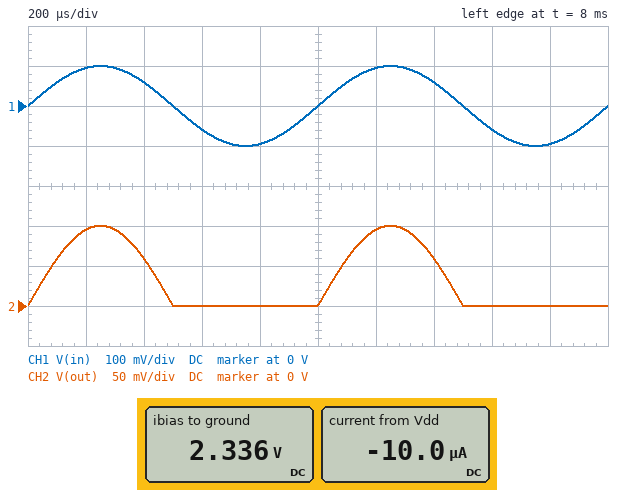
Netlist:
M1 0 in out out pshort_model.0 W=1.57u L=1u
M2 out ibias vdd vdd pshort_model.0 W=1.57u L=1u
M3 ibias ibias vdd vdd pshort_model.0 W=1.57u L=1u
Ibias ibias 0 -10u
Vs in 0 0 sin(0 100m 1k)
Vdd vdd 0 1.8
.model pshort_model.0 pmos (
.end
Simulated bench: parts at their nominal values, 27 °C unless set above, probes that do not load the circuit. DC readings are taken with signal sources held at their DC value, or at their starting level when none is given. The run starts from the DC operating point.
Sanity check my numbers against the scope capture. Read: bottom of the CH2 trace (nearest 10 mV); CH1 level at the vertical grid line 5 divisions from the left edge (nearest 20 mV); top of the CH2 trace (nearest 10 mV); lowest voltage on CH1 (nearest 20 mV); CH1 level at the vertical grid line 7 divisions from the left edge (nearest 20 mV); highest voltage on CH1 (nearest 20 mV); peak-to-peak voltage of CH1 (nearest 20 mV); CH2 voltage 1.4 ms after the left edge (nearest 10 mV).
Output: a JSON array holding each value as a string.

["0 V", "0 V", "100 mV", "-100 mV", "60 mV", "100 mV", "200 mV", "60 mV"]
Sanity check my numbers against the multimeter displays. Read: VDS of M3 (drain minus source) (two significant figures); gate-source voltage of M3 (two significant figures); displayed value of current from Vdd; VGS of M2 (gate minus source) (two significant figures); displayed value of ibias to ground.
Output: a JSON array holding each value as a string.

["540 mV", "540 mV", "-10.0 µA", "540 mV", "2.336 V"]
